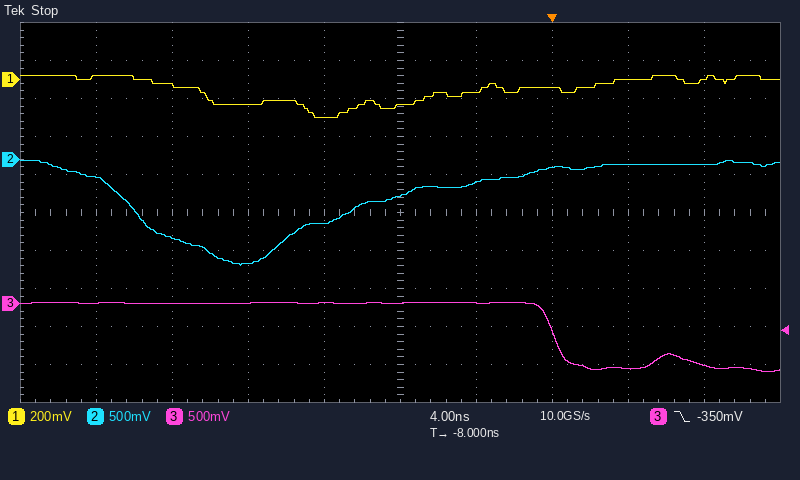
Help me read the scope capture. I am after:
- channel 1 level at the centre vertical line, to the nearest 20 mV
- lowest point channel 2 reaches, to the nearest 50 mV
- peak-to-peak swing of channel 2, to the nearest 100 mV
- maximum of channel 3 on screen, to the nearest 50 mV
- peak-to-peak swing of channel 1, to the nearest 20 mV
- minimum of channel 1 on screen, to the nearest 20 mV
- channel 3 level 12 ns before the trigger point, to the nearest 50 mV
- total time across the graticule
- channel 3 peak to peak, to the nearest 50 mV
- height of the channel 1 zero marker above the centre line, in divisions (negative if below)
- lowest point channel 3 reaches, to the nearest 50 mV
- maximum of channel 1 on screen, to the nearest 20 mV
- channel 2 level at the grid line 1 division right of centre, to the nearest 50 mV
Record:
-140 mV
-1.40 V
1.40 V
0 mV
220 mV
-200 mV
0 mV
40 ns
900 mV
+3.5 div
-900 mV
20 mV
-300 mV
